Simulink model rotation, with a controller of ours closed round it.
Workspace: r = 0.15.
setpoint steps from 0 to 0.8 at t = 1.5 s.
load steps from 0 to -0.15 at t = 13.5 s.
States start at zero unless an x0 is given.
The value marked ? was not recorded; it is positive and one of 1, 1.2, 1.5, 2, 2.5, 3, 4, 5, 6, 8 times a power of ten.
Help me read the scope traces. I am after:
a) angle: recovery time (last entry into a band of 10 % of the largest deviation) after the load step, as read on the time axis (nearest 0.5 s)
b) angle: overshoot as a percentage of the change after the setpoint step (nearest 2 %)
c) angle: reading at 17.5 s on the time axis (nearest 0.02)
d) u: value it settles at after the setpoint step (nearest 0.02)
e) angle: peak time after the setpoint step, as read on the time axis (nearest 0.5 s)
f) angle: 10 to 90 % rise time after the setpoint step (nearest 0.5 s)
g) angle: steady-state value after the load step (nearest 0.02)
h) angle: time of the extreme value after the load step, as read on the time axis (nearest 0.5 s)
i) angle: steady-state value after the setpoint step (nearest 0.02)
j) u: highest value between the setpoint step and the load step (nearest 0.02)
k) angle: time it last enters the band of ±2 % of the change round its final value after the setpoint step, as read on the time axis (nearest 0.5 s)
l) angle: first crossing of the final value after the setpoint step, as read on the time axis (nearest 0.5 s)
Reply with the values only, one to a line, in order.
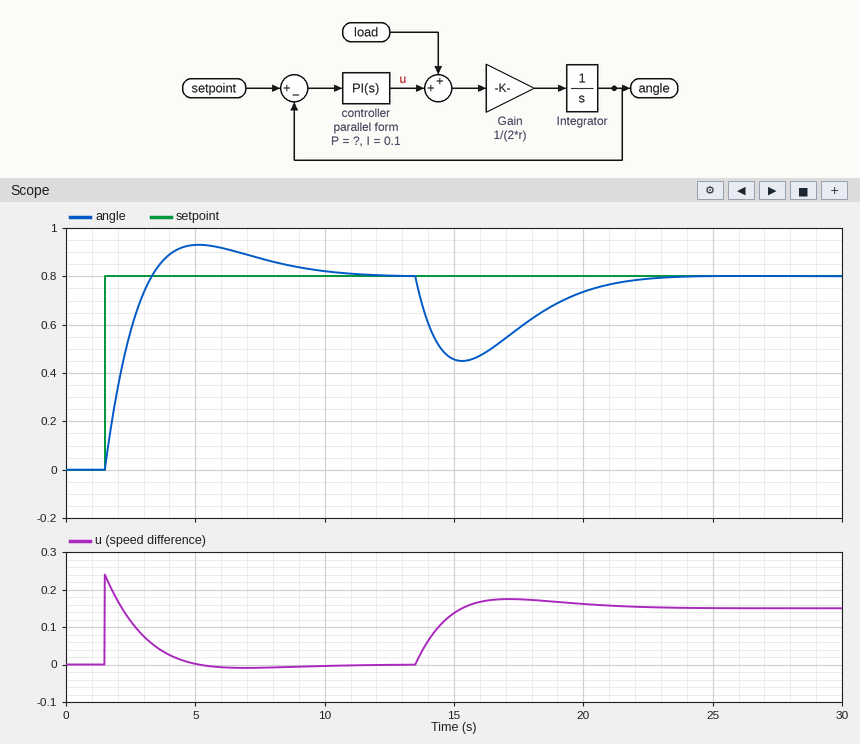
21.0 s
16 %
0.58
0.00
5.0 s
1.5 s
0.80
15.5 s
0.80
0.24
10.5 s
3.5 s
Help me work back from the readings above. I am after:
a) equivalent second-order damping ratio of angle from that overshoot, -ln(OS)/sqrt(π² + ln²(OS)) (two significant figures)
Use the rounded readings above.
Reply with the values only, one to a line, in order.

0.50
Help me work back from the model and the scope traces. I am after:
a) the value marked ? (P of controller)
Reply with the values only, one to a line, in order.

0.3
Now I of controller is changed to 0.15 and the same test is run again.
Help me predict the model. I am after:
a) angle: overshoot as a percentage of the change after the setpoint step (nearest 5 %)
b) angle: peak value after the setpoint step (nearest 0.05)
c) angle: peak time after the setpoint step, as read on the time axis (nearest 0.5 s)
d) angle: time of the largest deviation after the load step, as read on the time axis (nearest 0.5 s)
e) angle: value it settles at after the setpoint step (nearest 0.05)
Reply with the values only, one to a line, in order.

20 %
0.95
4.5 s
15.0 s
0.80
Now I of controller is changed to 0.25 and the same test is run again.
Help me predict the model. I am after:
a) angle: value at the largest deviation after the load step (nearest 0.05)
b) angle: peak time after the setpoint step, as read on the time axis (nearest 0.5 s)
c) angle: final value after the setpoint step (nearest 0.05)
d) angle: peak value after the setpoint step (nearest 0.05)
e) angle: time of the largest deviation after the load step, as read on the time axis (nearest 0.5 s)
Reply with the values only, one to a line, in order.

0.50
4.0 s
0.80
1.00
15.0 s
